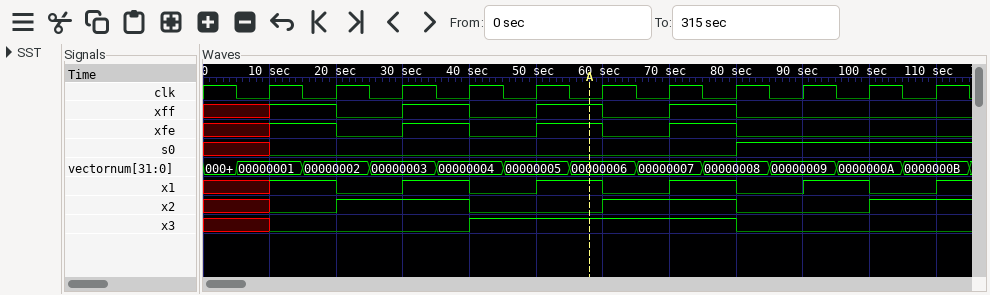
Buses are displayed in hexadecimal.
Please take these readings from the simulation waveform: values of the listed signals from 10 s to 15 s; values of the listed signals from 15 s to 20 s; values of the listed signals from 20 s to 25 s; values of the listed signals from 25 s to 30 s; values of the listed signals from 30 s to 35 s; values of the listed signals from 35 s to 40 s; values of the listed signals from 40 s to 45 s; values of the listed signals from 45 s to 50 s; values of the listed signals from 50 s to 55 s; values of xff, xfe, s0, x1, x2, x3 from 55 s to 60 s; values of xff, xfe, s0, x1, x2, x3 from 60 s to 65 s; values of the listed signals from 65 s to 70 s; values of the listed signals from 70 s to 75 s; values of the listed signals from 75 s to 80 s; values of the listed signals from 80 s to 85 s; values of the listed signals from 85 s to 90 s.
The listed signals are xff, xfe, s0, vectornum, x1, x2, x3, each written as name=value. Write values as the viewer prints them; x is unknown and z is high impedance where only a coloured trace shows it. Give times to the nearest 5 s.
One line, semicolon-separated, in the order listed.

xff=1, xfe=1, s0=0, vectornum=00000001, x1=1, x2=0, x3=0; xff=1, xfe=1, s0=0, vectornum=00000002, x1=1, x2=0, x3=0; xff=0, xfe=0, s0=0, vectornum=00000002, x1=0, x2=1, x3=0; xff=0, xfe=0, s0=0, vectornum=00000003, x1=0, x2=1, x3=0; xff=1, xfe=1, s0=0, vectornum=00000003, x1=1, x2=1, x3=0; xff=1, xfe=1, s0=0, vectornum=00000004, x1=1, x2=1, x3=0; xff=0, xfe=0, s0=0, vectornum=00000004, x1=0, x2=0, x3=1; xff=0, xfe=0, s0=0, vectornum=00000005, x1=0, x2=0, x3=1; xff=1, xfe=1, s0=0, vectornum=00000005, x1=1, x2=0, x3=1; xff=1, xfe=1, s0=0, x1=1, x2=0, x3=1; xff=0, xfe=0, s0=0, x1=0, x2=1, x3=1; xff=0, xfe=0, s0=0, vectornum=00000007, x1=0, x2=1, x3=1; xff=1, xfe=1, s0=0, vectornum=00000007, x1=1, x2=1, x3=1; xff=1, xfe=1, s0=0, vectornum=00000008, x1=1, x2=1, x3=1; xff=0, xfe=0, s0=1, vectornum=00000008, x1=0, x2=0, x3=0; xff=0, xfe=0, s0=1, vectornum=00000009, x1=0, x2=0, x3=0
